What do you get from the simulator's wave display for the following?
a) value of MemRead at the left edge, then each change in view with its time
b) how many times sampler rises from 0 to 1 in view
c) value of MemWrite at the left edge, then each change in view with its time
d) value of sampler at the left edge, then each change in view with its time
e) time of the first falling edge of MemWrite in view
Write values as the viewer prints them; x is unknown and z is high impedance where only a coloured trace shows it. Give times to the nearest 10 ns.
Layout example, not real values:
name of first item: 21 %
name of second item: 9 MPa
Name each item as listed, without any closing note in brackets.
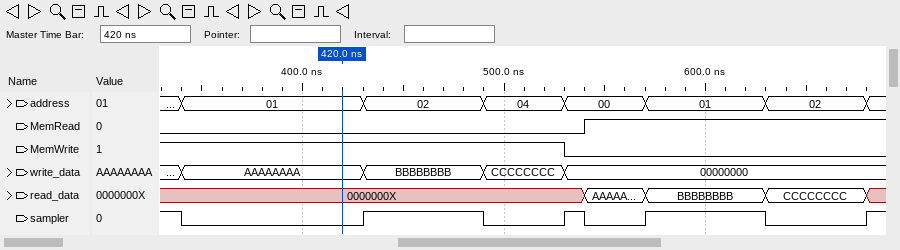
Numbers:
value of MemRead at the left edge, then each change in view with its time: 0, 1 at 540 ns
how many times sampler rises from 0 to 1 in view: 4
value of MemWrite at the left edge, then each change in view with its time: 1, 0 at 530 ns
value of sampler at the left edge, then each change in view with its time: 1, 0 at 340 ns, 1 at 430 ns, 0 at 490 ns, 1 at 530 ns, 0 at 540 ns, 1 at 570 ns, 0 at 630 ns, 1 at 680 ns
time of the first falling edge of MemWrite in view: 530 ns
